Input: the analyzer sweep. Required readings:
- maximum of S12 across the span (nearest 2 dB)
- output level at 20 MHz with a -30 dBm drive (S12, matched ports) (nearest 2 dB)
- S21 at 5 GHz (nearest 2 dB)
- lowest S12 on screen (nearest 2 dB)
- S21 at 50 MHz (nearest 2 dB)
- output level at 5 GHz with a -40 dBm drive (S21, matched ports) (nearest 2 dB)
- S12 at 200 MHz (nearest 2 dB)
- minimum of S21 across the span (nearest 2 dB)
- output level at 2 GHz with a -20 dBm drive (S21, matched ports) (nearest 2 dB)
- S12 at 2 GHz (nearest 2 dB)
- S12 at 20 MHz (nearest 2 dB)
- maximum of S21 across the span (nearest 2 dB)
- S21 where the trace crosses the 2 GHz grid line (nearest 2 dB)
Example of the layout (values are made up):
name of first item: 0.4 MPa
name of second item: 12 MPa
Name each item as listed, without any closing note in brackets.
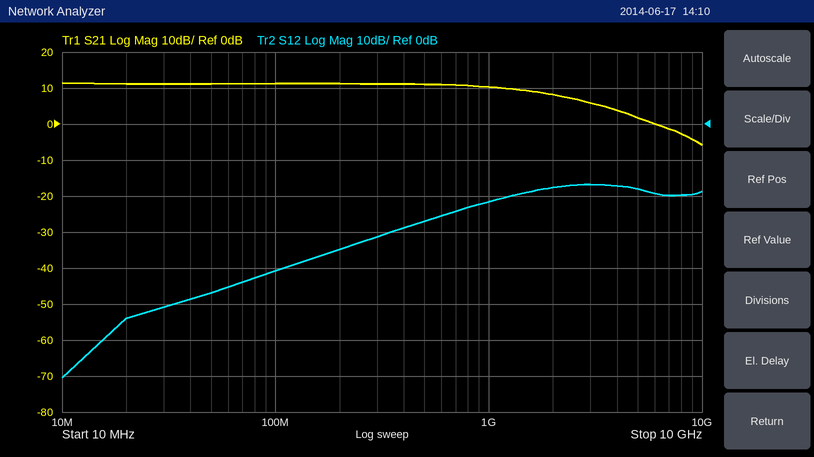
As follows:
maximum of S12 across the span: -16 dB
output level at 20 MHz with a -30 dBm drive (S12, matched ports): -84 dBm
S21 at 5 GHz: 2 dB
lowest S12 on screen: -70 dB
S21 at 50 MHz: 12 dB
output level at 5 GHz with a -40 dBm drive (S21, matched ports): -38 dBm
S12 at 200 MHz: -34 dB
minimum of S21 across the span: -6 dB
output level at 2 GHz with a -20 dBm drive (S21, matched ports): -12 dBm
S12 at 2 GHz: -18 dB
S12 at 20 MHz: -54 dB
maximum of S21 across the span: 12 dB
S21 where the trace crosses the 2 GHz grid line: 8 dB
